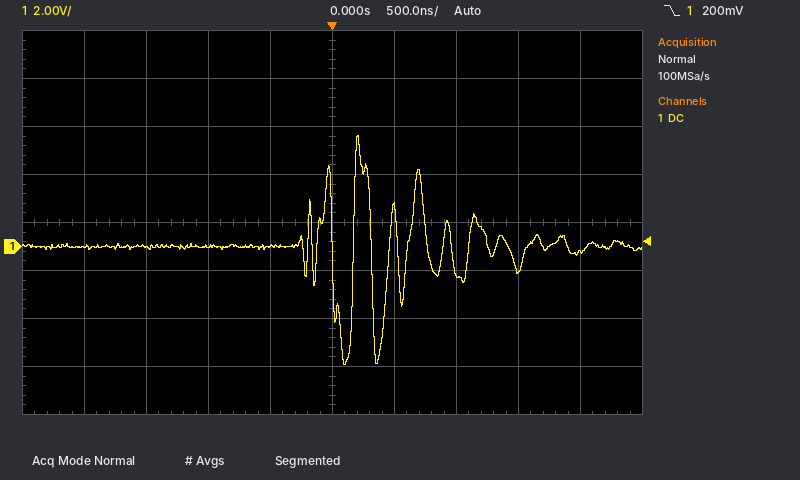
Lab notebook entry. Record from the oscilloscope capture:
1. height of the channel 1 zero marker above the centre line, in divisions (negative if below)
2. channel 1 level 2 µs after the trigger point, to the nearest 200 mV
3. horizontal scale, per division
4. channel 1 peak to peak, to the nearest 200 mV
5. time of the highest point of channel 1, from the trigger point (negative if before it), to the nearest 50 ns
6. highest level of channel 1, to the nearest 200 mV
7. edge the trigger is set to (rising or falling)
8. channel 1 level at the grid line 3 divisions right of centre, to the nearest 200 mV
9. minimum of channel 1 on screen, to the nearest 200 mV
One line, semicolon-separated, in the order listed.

-0.5 div; -200 mV; 500 ns; 9.6 V; +200 ns; 4.6 V; falling; -1.0 V; -5.0 V
